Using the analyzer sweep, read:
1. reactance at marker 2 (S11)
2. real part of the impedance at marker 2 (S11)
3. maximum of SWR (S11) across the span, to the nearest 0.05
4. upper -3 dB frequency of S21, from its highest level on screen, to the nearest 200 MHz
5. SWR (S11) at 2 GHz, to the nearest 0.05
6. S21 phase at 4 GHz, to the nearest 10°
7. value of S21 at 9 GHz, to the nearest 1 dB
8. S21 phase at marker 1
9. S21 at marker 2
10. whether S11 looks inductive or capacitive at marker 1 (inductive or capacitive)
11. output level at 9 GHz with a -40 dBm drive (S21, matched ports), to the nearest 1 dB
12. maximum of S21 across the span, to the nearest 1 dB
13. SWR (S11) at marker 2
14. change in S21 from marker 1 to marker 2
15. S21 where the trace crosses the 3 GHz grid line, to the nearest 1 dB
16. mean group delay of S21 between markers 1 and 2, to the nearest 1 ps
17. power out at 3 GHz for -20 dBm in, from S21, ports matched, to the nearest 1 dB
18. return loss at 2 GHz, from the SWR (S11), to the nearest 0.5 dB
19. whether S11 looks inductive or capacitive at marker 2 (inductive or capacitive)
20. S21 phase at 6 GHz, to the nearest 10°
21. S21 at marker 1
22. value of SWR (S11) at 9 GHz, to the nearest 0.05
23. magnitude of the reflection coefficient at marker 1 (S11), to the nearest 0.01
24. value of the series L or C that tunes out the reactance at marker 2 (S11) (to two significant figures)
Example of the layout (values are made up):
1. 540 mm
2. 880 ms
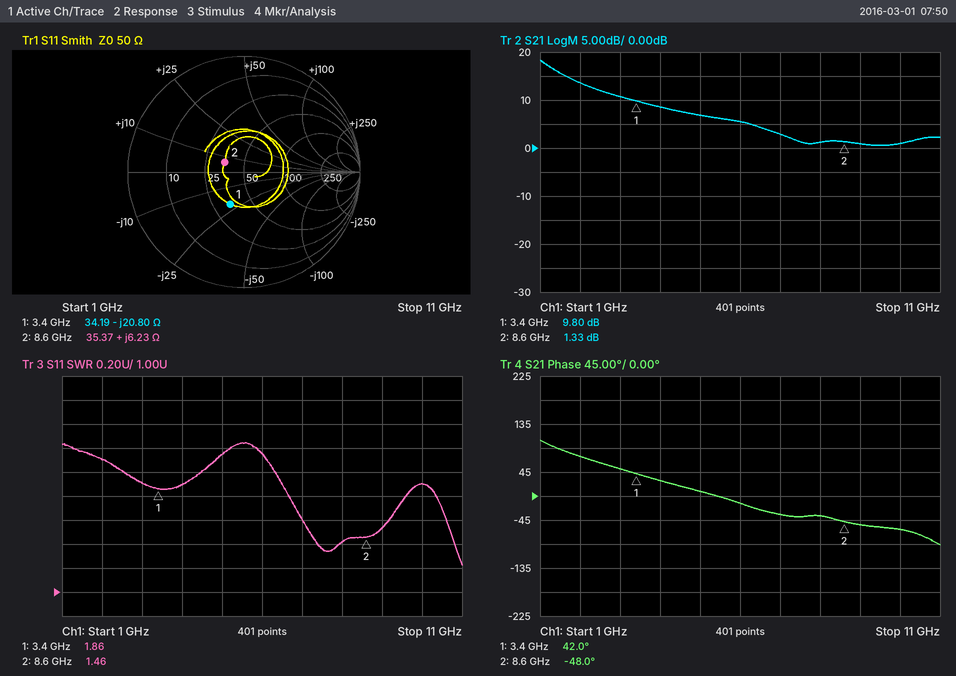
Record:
1. +6.23 Ω
2. 35.37 Ω
3. 2.25
4. 1.6 GHz
5. 2.10
6. 30°
7. 1 dB
8. 42.0°
9. 1.33 dB
10. capacitive
11. -39 dBm
12. 18 dB
13. 1.46
14. -8.47 dB
15. 11 dB
16. 48 ps
17. -9 dBm
18. 9.0 dB
19. inductive
20. -10°
21. 9.80 dB
22. 1.55
23. 0.30
24. 3.0 pF
